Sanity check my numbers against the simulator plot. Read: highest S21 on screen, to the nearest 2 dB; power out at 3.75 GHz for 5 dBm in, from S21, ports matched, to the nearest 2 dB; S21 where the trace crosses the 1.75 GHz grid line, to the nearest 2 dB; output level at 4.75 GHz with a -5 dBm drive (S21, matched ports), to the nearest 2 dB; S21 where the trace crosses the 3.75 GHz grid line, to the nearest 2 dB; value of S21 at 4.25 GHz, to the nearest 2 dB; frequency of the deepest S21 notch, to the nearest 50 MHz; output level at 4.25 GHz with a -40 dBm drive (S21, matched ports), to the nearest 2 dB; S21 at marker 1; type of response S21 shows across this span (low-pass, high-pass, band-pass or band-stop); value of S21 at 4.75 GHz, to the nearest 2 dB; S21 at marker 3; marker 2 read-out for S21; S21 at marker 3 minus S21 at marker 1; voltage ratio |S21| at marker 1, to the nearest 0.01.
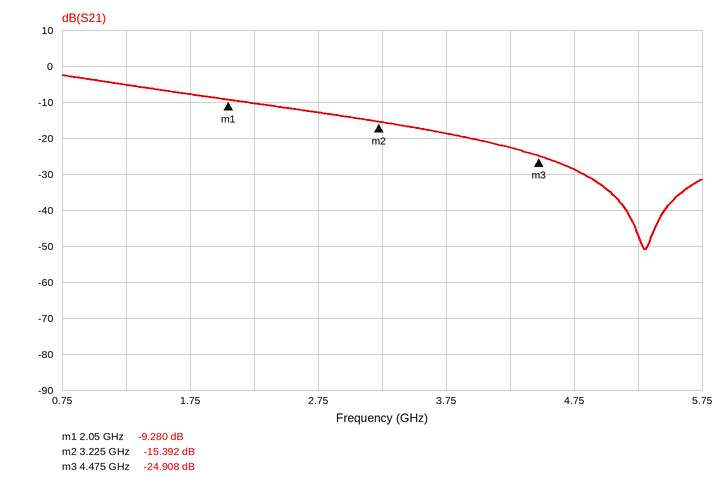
-2 dB
-14 dBm
-8 dB
-34 dBm
-18 dB
-22 dB
5.30 GHz
-62 dBm
-9.280 dB
low-pass
-28 dB
-24.908 dB
-15.392 dB
-15.628 dB
0.34
